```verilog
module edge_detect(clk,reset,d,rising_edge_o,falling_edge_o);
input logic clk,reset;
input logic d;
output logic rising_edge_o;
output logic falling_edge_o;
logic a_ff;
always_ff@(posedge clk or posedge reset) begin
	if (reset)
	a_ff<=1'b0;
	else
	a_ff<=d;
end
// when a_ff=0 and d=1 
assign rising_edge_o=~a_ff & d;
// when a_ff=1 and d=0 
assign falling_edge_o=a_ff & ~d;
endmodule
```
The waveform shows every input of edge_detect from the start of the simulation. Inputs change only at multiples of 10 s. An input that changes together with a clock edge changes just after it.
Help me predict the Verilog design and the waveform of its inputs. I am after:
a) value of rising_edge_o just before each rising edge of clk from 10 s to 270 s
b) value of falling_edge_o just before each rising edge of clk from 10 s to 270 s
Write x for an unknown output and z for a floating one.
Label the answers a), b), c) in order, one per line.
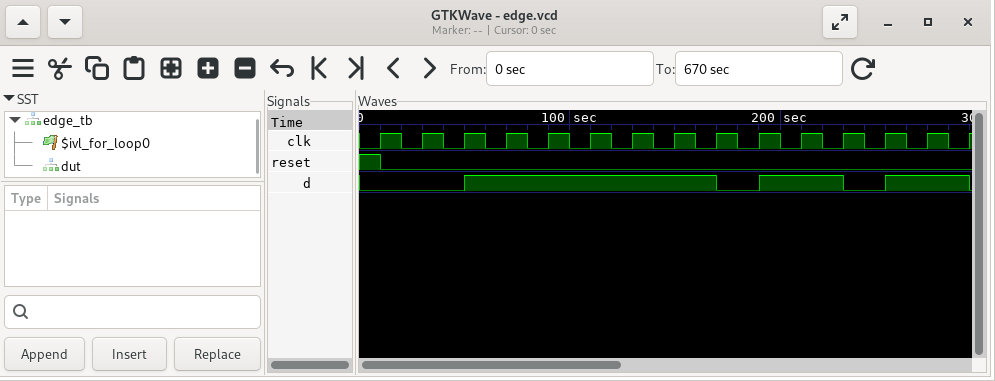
a) 0 0 0 1 0 0 0 0 0 0 1 0 0 1
b) 0 0 0 0 0 0 0 0 0 1 0 0 1 0
